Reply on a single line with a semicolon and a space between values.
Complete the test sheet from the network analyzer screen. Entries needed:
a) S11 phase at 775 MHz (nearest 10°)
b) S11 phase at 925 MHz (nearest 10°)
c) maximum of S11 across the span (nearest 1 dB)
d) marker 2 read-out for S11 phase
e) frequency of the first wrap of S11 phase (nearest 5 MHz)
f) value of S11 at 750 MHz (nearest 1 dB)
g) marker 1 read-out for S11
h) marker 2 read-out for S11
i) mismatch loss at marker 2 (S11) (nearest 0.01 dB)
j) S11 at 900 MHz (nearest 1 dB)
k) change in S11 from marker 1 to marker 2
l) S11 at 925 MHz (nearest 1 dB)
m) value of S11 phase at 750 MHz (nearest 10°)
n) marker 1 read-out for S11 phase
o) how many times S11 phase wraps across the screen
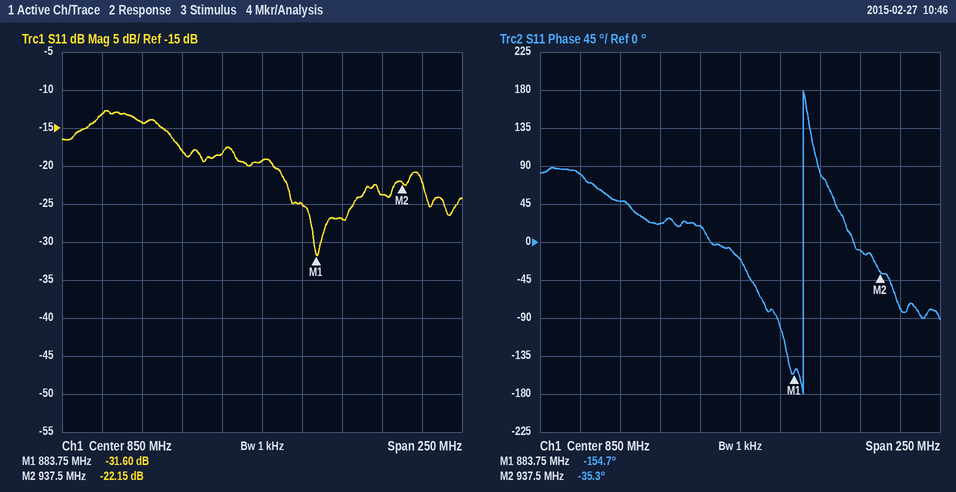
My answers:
50°; -10°; -13 dB; -35.3°; 890 MHz; -13 dB; -31.60 dB; -22.15 dB; 0.03 dB; -27 dB; 9.45 dB; -24 dB; 80°; -154.7°; 1
